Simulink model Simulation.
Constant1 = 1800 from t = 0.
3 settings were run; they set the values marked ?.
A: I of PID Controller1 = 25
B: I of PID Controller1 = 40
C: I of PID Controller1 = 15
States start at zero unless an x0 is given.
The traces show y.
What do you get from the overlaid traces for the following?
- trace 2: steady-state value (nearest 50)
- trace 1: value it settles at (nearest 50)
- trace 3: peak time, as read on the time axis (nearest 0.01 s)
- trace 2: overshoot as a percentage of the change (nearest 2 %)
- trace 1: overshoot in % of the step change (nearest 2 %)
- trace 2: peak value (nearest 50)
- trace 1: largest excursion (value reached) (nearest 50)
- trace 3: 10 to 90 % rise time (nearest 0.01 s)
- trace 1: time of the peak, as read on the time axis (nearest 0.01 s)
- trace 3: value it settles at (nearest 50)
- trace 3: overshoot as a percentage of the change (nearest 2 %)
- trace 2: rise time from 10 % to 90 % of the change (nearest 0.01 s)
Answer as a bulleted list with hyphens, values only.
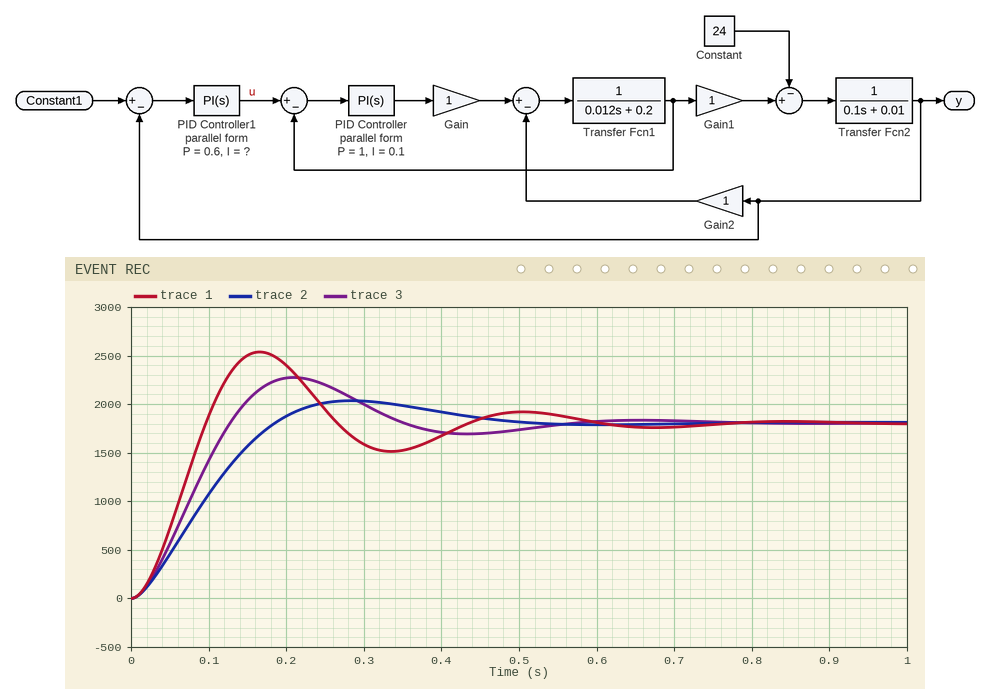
- 1800
- 1800
- 0.21 s
- 12 %
- 40 %
- 2050
- 2550
- 0.09 s
- 0.17 s
- 1800
- 26 %
- 0.13 s
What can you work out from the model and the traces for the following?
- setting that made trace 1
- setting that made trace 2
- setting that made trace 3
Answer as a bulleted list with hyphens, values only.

- B
- C
- A
